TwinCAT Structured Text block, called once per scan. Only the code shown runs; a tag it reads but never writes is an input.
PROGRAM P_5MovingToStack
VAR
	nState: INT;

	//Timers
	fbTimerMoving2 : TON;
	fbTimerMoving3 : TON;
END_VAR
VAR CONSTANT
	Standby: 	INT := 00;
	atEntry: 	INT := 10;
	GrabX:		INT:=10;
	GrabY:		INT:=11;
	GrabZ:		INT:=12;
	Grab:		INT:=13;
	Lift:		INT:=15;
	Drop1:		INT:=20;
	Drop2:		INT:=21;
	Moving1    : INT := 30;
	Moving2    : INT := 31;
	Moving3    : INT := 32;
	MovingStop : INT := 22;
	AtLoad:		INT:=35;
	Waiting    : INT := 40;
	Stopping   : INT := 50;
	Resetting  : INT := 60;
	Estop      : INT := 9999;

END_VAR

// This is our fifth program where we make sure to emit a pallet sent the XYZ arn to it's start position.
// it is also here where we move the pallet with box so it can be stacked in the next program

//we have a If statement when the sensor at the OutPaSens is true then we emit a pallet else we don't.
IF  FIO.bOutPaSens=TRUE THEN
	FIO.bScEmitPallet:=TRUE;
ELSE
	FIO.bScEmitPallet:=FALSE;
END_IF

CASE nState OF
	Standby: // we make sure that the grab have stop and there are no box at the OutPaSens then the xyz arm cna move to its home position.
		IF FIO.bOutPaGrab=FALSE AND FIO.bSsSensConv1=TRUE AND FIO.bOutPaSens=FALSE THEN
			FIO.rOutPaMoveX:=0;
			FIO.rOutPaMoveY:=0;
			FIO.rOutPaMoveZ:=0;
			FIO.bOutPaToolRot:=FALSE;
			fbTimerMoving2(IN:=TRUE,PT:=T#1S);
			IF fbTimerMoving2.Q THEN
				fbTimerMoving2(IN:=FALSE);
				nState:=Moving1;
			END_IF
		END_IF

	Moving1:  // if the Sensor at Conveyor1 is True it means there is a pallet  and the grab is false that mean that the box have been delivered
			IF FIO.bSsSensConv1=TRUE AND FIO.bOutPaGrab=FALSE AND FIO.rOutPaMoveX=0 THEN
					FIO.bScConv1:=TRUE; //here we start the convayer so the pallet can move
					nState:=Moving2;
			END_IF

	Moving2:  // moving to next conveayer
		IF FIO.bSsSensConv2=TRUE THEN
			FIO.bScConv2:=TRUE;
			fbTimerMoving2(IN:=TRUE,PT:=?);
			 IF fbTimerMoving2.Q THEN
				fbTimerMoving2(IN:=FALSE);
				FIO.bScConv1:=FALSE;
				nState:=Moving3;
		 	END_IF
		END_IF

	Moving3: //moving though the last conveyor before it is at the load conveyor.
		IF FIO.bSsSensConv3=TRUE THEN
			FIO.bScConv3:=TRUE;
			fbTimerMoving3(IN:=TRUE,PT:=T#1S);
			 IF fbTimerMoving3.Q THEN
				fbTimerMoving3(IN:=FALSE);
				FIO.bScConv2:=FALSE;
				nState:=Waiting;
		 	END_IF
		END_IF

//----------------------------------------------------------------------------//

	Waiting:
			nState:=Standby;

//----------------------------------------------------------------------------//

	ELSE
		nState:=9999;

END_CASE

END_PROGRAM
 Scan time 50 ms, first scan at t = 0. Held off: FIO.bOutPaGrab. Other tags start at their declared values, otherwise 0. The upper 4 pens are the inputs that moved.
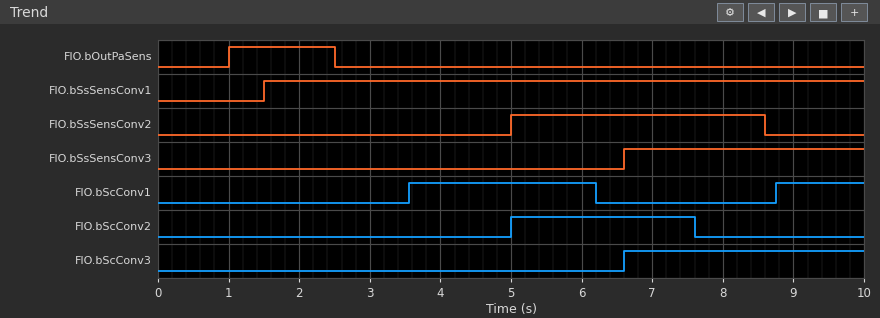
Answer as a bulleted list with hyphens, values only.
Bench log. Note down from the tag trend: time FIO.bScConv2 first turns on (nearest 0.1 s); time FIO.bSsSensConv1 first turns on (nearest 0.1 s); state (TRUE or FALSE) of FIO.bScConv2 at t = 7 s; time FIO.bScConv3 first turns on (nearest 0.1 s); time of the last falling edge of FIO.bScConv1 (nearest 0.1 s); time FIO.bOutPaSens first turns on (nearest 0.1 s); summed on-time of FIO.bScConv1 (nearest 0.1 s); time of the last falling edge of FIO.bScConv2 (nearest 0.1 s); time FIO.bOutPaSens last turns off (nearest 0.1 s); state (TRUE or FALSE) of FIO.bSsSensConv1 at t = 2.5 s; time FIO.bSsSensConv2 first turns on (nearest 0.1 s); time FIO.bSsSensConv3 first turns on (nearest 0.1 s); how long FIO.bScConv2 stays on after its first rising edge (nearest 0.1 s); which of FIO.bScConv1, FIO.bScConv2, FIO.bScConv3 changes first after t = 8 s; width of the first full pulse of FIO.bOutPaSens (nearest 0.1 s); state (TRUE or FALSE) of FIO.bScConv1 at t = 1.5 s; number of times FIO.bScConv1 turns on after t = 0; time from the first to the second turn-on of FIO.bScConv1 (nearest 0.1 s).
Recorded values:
- 5.0 s
- 1.5 s
- TRUE
- 6.6 s
- 6.2 s
- 1.0 s
- 3.9 s
- 7.6 s
- 2.5 s
- TRUE
- 5.0 s
- 6.6 s
- 2.6 s
- FIO.bScConv1
- 1.5 s
- FALSE
- 2
- 5.2 s
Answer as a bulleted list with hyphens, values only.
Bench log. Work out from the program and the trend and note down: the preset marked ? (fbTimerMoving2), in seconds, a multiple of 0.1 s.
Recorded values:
- 1.2 s
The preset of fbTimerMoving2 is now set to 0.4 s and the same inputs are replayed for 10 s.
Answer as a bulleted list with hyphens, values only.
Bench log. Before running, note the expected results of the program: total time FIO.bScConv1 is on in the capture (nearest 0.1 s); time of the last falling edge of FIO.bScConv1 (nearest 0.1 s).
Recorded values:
- 3.1 s
- 5.4 s
